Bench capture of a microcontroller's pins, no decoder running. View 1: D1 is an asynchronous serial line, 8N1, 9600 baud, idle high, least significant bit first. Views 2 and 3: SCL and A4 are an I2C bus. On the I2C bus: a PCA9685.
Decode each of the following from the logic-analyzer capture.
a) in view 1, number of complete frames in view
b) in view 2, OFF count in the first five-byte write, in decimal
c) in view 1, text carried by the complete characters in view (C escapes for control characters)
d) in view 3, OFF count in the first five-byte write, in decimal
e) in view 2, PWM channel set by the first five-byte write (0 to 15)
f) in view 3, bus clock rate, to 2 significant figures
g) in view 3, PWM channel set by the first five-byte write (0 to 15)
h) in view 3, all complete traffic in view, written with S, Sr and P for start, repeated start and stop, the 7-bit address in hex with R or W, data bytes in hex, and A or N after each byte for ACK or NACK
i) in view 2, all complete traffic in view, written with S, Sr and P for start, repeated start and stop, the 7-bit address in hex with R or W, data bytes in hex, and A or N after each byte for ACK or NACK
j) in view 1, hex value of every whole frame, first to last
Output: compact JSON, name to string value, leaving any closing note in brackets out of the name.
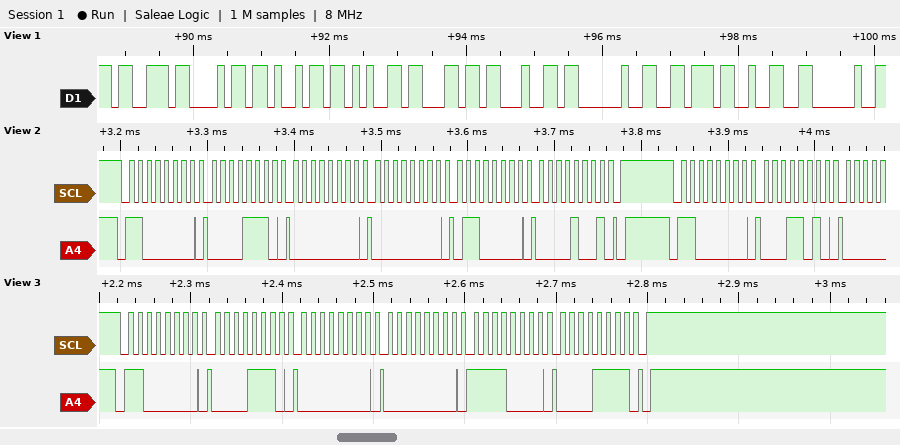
{"in view 1, number of complete frames in view": "10", "in view 2, OFF count in the first five-byte write, in decimal": "2400", "in view 1, text carried by the complete characters in view": "\"shield v2 \"", "in view 3, OFF count in the first five-byte write, in decimal": "4080", "in view 2, PWM channel set by the first five-byte write": "2", "in view 3, bus clock rate, to 2 significant figures": "100 kHz", "in view 3, PWM channel set by the first five-byte write": "2", "in view 3, all complete traffic in view, written with S, Sr and P for start, repeated start and stop, the 7-bit address in hex with R or W, data bytes in hex, and A or N after each byte for ACK or NACK": "S 60W A 0E A 00 A 00 A F0 A 0F A P", "in view 2, all complete traffic in view, written with S, Sr and P for start, repeated start and stop, the 7-bit address in hex with R or W, data bytes in hex, and A or N after each byte for ACK or NACK": "S 60W A 0E A 00 A 00 A 60 A 09 A P S 60W A 1A A", "in view 1, hex value of every whole frame, first to last": "73 68 69 65 6C 64 20 76 32 20"}
